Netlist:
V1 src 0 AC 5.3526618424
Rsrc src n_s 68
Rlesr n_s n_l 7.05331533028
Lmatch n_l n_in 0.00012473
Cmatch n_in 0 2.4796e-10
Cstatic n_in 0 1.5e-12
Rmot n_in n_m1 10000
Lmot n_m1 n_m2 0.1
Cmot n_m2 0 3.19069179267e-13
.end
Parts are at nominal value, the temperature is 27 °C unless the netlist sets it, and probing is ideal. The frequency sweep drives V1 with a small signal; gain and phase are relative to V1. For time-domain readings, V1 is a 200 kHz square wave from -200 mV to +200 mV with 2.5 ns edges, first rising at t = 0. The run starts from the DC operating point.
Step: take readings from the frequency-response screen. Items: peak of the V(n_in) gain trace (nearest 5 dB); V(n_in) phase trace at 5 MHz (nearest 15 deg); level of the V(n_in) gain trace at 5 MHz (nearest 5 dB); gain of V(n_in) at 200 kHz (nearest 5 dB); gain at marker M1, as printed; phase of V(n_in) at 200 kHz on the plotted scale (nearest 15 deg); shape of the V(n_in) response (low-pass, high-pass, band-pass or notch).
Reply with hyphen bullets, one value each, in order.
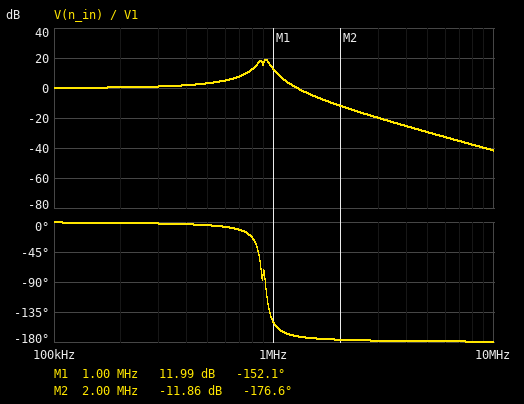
- 20 dB
- -180 deg
- -30 dB
- 0 dB
- 11.99 dB
- 0 deg
- low-pass
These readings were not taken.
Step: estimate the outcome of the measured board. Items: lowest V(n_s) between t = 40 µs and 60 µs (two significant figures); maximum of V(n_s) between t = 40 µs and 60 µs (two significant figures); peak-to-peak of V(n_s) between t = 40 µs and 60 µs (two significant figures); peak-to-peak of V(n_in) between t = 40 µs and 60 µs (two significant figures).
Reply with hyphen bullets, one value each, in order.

- -230 mV
- 230 mV
- 450 mV
- 1.0 V
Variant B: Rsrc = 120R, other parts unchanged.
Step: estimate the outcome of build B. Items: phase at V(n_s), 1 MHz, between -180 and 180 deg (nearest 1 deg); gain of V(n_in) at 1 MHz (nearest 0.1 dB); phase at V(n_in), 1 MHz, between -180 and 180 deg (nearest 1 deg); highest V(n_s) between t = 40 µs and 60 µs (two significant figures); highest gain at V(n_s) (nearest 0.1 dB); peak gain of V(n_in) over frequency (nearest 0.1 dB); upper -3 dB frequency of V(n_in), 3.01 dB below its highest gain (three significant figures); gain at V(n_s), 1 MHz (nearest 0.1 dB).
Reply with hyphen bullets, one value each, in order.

- 39 deg
- 10.5 dB
- -138 deg
- 240 mV
- 0 dB
- 14.6 dB
- 981 kHz
- -2.5 dB
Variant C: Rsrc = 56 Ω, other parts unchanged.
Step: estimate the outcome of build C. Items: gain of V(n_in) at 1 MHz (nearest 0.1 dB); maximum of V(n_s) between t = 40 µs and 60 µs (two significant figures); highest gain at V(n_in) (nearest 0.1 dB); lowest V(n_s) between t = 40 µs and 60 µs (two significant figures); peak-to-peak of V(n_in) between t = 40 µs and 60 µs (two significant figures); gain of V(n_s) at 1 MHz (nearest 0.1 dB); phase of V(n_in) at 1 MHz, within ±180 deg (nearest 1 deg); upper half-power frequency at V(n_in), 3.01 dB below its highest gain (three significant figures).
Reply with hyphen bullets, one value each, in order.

- 12.3 dB
- 220 mV
- 20.4 dB
- -220 mV
- 1.0 V
- -0.8 dB
- -156 deg
- 950 kHz
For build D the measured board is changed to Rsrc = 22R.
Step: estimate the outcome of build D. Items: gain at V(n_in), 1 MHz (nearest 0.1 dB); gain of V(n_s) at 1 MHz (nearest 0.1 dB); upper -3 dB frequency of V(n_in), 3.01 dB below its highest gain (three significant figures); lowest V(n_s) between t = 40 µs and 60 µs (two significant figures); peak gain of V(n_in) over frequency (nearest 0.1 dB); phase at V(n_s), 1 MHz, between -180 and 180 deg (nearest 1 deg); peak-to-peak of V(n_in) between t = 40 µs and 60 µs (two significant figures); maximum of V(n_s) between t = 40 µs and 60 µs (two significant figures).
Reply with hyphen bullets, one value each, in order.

- 12.9 dB
- -0.2 dB
- 932 kHz
- -210 mV
- 26.3 dB
- 9 deg
- 1.0 V
- 210 mV
